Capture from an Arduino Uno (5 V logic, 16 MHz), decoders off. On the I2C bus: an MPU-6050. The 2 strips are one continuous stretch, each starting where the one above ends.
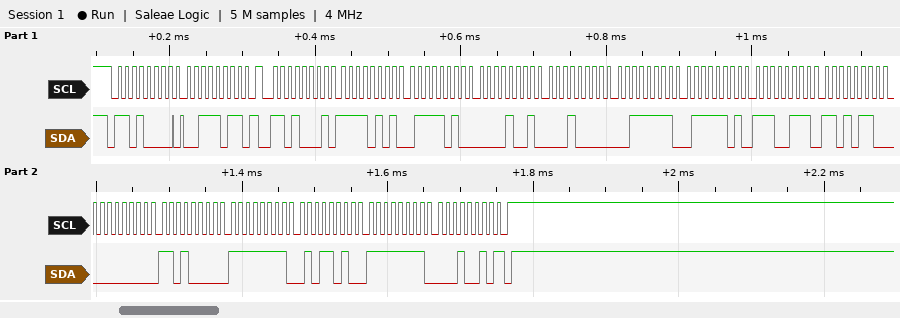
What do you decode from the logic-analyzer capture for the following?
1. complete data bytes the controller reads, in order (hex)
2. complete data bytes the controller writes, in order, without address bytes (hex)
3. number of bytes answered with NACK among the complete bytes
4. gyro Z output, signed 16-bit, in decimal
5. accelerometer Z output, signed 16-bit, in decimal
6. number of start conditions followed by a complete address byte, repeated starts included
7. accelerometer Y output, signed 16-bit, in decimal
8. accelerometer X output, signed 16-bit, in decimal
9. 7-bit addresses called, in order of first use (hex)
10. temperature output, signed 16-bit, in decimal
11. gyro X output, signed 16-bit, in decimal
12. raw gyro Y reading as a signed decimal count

F5 7A 09 10 3F 7D E7 D6 00 D0 FF 5A FF 12
3B
1
-238
16253
2
2320
-2694
0x68
-6186
208
-166
